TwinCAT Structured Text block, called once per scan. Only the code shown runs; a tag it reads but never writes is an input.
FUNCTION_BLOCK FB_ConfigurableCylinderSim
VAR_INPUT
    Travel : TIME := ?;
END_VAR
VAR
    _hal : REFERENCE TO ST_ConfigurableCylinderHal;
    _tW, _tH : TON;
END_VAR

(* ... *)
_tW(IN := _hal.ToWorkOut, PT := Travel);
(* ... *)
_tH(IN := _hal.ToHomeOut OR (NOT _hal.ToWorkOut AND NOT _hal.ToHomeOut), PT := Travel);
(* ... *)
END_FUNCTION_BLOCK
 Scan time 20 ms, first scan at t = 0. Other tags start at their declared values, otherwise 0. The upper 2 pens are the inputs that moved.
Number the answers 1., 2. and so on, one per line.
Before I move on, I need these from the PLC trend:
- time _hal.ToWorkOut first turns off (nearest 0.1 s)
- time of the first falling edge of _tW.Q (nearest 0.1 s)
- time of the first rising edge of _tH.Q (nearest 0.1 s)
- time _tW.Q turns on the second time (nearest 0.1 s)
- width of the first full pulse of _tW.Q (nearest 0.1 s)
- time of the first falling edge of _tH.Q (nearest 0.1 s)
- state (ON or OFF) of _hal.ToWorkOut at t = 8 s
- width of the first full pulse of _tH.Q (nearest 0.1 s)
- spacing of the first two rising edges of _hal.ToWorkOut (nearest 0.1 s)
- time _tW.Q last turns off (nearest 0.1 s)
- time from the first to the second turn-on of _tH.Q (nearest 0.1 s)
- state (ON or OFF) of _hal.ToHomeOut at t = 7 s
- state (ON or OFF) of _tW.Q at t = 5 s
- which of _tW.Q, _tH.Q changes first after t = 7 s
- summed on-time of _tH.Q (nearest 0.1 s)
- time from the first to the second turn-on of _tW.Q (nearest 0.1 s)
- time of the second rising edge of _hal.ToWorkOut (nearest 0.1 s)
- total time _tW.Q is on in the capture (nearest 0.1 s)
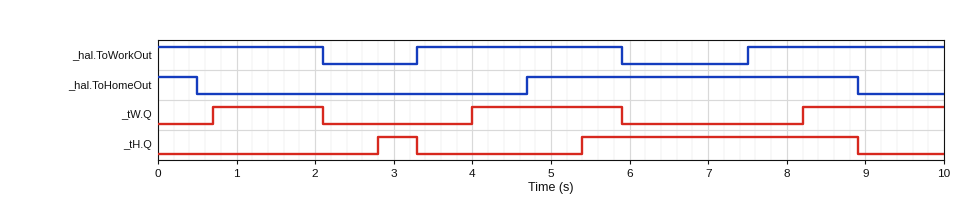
1. 2.1 s
2. 2.1 s
3. 2.8 s
4. 4.0 s
5. 1.4 s
6. 3.3 s
7. ON
8. 0.5 s
9. 4.2 s
10. 5.9 s
11. 2.6 s
12. ON
13. ON
14. _tW.Q
15. 4.0 s
16. 3.3 s
17. 7.5 s
18. 5.1 s
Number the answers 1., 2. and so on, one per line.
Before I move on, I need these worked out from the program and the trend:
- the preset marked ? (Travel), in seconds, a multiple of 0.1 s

1. 0.7 s
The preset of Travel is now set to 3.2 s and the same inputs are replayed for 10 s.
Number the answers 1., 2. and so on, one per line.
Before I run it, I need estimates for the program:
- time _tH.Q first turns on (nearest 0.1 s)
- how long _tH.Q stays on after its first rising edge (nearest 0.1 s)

1. 7.9 s
2. 1.0 s
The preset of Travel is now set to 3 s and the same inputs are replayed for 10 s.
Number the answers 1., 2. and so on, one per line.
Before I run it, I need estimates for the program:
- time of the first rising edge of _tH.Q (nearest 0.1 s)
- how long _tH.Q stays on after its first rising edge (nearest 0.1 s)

1. 7.7 s
2. 1.2 s
